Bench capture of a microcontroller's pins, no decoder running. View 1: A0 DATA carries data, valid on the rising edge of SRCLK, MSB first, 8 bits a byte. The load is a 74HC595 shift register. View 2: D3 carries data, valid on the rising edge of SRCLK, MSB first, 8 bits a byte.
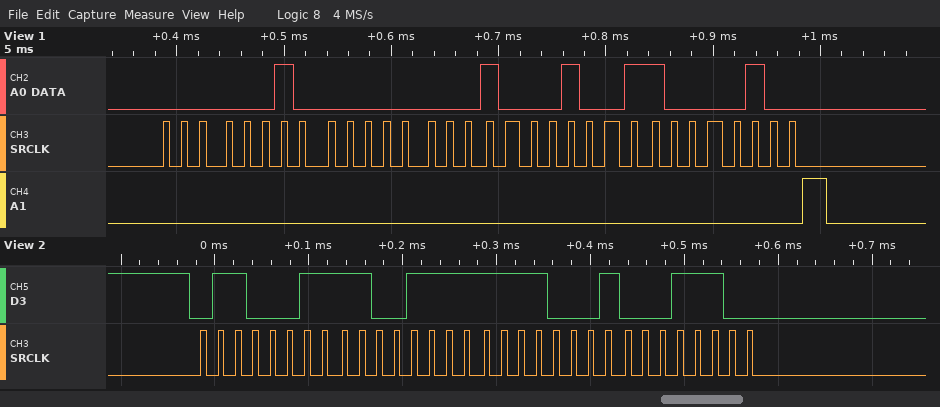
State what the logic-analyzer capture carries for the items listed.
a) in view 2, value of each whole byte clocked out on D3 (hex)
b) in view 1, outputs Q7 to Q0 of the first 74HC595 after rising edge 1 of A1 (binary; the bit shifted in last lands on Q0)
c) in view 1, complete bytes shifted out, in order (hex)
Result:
63 CF F1 1C
10000100
0x02 0x00 0x89 0x84
